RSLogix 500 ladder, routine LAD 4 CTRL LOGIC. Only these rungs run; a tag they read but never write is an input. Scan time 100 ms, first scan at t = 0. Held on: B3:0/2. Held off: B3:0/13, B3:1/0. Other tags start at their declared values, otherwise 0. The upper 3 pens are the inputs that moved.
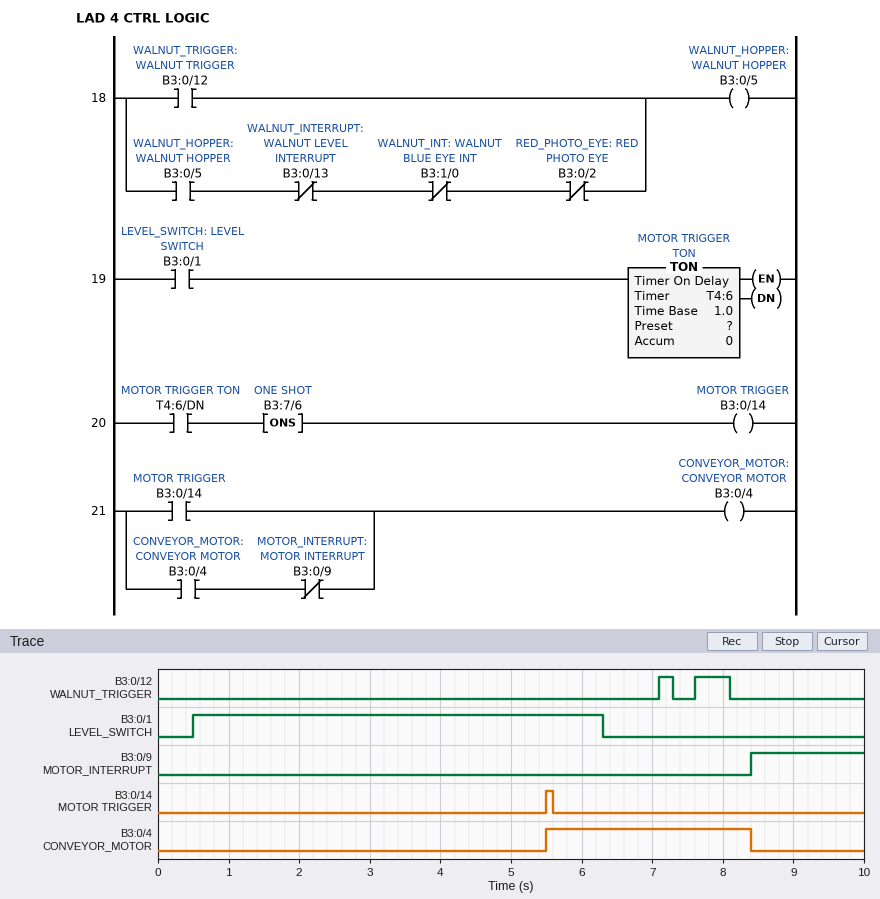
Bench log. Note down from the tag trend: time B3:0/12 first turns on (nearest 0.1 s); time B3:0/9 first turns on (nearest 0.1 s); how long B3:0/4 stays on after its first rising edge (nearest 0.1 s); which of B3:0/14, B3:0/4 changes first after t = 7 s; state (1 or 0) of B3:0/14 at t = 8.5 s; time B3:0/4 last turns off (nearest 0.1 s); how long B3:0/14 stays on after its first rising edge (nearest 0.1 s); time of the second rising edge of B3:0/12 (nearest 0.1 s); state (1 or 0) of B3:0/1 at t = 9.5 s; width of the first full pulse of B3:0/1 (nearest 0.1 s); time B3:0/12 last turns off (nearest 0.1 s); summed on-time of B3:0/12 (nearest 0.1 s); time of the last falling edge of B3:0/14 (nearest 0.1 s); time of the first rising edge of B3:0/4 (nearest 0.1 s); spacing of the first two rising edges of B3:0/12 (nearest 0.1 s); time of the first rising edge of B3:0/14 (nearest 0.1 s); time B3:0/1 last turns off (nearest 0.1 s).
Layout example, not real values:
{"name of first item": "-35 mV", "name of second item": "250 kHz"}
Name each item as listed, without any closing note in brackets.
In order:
{"time B3:0/12 first turns on": "7.1 s", "time B3:0/9 first turns on": "8.4 s", "how long B3:0/4 stays on after its first rising edge": "2.9 s", "which of B3:0/14, B3:0/4 changes first after t = 7 s": "B3:0/4", "state (1 or 0) of B3:0/14 at t = 8.5 s": "0", "time B3:0/4 last turns off": "8.4 s", "how long B3:0/14 stays on after its first rising edge": "0.1 s", "time of the second rising edge of B3:0/12": "7.6 s", "state (1 or 0) of B3:0/1 at t = 9.5 s": "0", "width of the first full pulse of B3:0/1": "5.8 s", "time B3:0/12 last turns off": "8.1 s", "summed on-time of B3:0/12": "0.7 s", "time of the last falling edge of B3:0/14": "5.6 s", "time of the first rising edge of B3:0/4": "5.5 s", "spacing of the first two rising edges of B3:0/12": "0.5 s", "time of the first rising edge of B3:0/14": "5.5 s", "time B3:0/1 last turns off": "6.3 s"}
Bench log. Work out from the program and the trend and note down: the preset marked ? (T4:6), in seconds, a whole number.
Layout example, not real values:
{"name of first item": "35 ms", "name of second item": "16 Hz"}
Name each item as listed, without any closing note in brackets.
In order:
{"the preset marked ? (T4:6), in seconds, a whole number": "5 s"}
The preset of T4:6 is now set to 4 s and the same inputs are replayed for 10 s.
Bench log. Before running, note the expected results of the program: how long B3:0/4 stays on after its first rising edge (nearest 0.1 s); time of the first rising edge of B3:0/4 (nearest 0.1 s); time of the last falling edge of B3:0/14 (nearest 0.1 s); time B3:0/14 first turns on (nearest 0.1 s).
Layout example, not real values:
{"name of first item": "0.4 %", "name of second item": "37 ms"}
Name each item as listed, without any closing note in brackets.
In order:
{"how long B3:0/4 stays on after its first rising edge": "3.9 s", "time of the first rising edge of B3:0/4": "4.5 s", "time of the last falling edge of B3:0/14": "4.6 s", "time B3:0/14 first turns on": "4.5 s"}
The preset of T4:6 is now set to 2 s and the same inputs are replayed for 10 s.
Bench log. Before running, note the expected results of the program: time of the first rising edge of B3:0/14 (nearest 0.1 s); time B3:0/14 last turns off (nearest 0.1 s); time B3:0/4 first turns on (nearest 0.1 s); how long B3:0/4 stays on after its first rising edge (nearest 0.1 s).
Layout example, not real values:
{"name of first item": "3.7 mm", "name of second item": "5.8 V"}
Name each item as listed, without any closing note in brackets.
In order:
{"time of the first rising edge of B3:0/14": "2.5 s", "time B3:0/14 last turns off": "2.6 s", "time B3:0/4 first turns on": "2.5 s", "how long B3:0/4 stays on after its first rising edge": "5.9 s"}
